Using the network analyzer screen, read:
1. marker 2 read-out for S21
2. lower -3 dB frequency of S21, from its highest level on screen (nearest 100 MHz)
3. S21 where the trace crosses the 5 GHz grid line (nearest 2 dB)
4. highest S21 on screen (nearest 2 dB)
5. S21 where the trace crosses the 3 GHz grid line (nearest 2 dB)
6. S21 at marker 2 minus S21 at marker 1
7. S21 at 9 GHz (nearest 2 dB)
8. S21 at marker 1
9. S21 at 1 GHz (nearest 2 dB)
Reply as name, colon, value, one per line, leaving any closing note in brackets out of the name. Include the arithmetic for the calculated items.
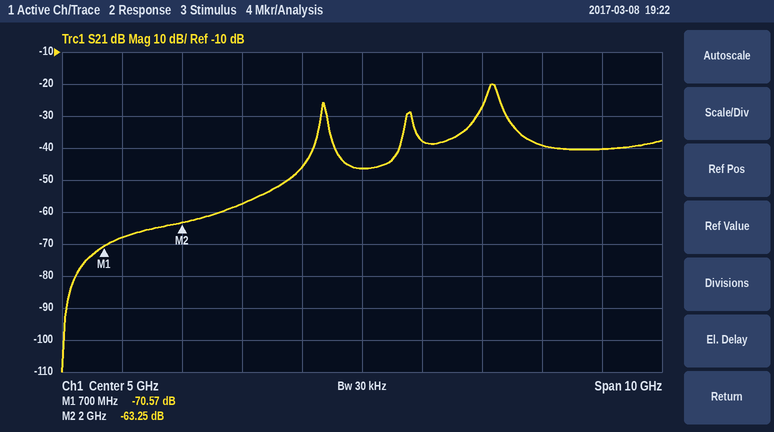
marker 2 read-out for S21: -63.25 dB
lower -3 dB frequency of S21, from its highest level on screen: 7.1 GHz
S21 where the trace crosses the 5 GHz grid line: -46 dB
highest S21 on screen: -20 dB
S21 where the trace crosses the 3 GHz grid line: -58 dB
S21 at marker 2 minus S21 at marker 1: -63.25 − (-70.57) = 7.32 dB
S21 at 9 GHz: -40 dB
S21 at marker 1: -70.57 dB
S21 at 1 GHz: -68 dB
